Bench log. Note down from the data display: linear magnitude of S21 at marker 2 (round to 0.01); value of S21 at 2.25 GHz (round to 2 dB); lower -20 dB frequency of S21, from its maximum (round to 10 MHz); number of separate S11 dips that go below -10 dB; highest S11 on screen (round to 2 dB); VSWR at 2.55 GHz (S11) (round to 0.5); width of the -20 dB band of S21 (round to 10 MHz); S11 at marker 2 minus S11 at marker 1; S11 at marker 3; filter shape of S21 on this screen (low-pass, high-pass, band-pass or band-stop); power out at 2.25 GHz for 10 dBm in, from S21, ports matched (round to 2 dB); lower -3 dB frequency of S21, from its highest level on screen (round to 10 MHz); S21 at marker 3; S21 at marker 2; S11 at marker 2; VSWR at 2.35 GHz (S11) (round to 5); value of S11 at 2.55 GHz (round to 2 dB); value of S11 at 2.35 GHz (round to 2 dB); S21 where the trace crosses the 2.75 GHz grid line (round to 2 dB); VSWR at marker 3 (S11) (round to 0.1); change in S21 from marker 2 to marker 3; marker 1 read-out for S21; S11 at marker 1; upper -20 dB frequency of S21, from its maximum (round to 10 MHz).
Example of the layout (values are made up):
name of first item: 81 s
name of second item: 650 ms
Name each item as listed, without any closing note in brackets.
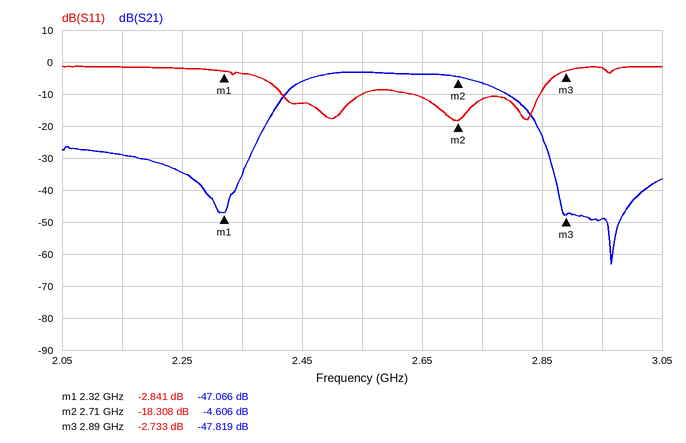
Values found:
linear magnitude of S21 at marker 2: 0.59
value of S21 at 2.25 GHz: -34 dB
lower -20 dB frequency of S21, from its maximum: 2.38 GHz
number of separate S11 dips that go below -10 dB: 3
highest S11 on screen: -2 dB
VSWR at 2.55 GHz (S11): 2.0
width of the -20 dB band of S21: 470 MHz
S11 at marker 2 minus S11 at marker 1: -15.467 dB
S11 at marker 3: -2.733 dB
filter shape of S21 on this screen: band-pass
power out at 2.25 GHz for 10 dBm in, from S21, ports matched: -24 dBm
lower -3 dB frequency of S21, from its highest level on screen: 2.45 GHz
S21 at marker 3: -47.819 dB
S21 at marker 2: -4.606 dB
S11 at marker 2: -18.308 dB
VSWR at 2.35 GHz (S11): 5
value of S11 at 2.55 GHz: -10 dB
value of S11 at 2.35 GHz: -4 dB
S21 where the trace crosses the 2.75 GHz grid line: -6 dB
VSWR at marker 3 (S11): 6.4
change in S21 from marker 2 to marker 3: -43.213 dB
marker 1 read-out for S21: -47.066 dB
S11 at marker 1: -2.841 dB
upper -20 dB frequency of S21, from its maximum: 2.85 GHz
